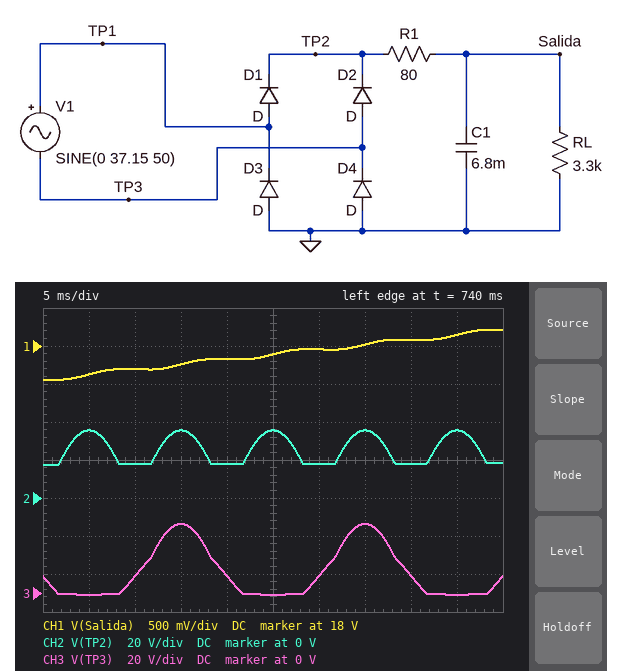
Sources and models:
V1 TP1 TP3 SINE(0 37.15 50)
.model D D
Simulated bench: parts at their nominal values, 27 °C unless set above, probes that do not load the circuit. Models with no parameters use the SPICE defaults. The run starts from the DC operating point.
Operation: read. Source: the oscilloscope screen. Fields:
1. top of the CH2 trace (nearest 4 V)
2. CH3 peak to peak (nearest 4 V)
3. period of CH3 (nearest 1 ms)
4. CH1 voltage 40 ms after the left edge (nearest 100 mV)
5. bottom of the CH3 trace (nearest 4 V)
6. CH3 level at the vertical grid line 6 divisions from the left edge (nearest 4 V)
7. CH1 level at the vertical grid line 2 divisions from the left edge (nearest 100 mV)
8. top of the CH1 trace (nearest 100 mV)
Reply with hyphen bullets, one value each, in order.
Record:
- 36 V
- 36 V
- 20 ms
- 18.1 V
- 0 V
- 8 V
- 17.7 V
- 18.2 V
